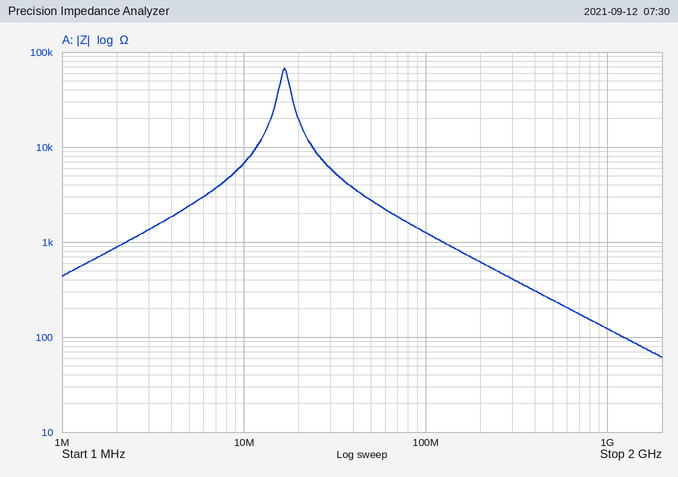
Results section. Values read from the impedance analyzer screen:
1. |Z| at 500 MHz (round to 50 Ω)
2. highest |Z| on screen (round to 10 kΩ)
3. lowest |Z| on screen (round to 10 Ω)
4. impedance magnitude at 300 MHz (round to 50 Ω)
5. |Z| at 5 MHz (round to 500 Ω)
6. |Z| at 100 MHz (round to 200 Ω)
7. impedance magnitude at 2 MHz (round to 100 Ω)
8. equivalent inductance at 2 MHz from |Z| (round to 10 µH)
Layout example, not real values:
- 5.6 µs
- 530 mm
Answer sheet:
- 250 Ω
- 70 kΩ
- 60 Ω
- 400 Ω
- 2.5 kΩ
- 1.2 kΩ
- 900 Ω
- 70 µH
